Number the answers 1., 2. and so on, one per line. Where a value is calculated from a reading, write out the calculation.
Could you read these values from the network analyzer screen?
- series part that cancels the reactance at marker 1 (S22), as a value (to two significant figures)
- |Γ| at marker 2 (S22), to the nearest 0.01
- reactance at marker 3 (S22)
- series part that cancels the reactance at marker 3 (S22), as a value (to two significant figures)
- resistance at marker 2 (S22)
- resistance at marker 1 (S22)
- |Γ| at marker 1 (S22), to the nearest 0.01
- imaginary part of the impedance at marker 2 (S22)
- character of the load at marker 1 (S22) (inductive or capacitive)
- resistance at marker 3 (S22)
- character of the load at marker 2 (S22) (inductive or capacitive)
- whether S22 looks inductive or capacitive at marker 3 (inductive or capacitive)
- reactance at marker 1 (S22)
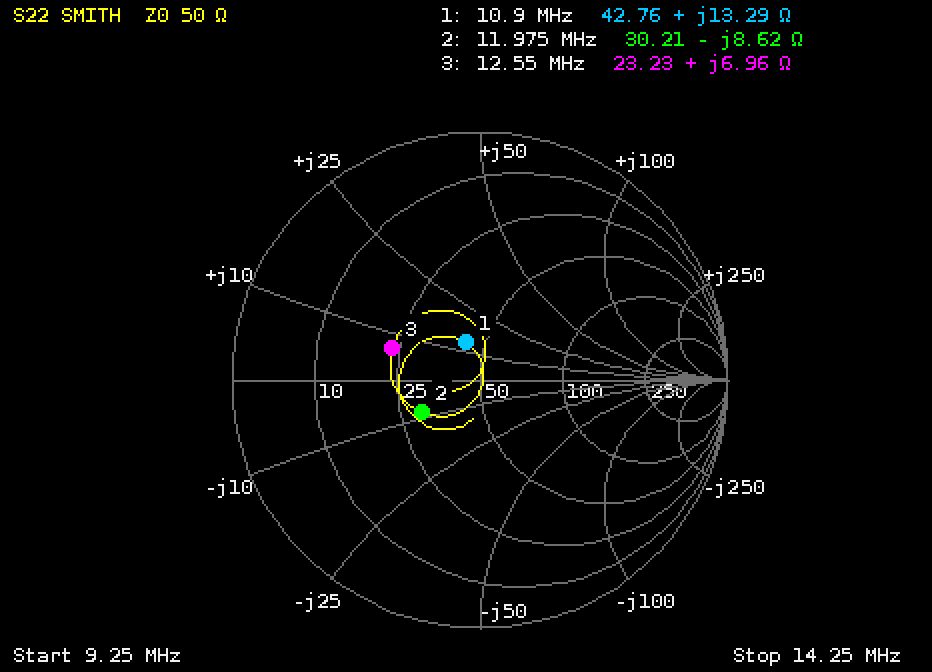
1. C = 1/(2π × 10.9 MHz × 13.29 Ω) ≈ 1.1 nF
2. 0.27
3. +6.96 Ω
4. C = 1/(2π × 12.55 MHz × 6.96 Ω) ≈ 1.8 nF
5. 30.21 Ω
6. 42.76 Ω
7. 0.16
8. -8.62 Ω
9. inductive
10. 23.23 Ω
11. capacitive
12. inductive
13. +13.29 Ω
